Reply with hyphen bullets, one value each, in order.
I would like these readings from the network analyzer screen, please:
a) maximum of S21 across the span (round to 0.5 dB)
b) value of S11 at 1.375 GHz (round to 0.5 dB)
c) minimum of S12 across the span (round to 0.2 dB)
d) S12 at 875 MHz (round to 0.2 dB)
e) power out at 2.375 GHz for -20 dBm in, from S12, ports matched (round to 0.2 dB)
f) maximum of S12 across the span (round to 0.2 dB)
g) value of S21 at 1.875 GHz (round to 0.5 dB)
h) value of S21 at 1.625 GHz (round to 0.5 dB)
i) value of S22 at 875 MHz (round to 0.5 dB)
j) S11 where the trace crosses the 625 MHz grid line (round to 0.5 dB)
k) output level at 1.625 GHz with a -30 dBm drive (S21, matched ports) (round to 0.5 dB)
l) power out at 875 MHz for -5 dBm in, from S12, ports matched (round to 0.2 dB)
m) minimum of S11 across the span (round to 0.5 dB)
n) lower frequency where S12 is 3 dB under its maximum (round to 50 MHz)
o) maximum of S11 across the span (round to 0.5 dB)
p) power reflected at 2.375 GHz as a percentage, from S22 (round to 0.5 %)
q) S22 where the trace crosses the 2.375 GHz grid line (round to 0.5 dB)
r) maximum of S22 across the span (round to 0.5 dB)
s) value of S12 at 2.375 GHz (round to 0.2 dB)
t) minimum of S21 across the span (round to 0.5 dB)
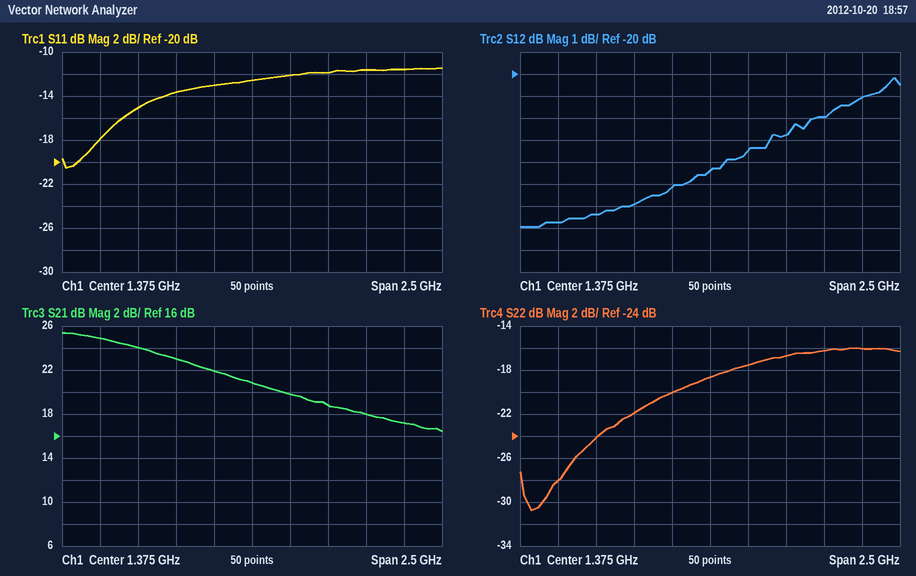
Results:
- 25.5 dB
- -12.5 dB
- -27.0 dB
- -26.0 dB
- -41.0 dBm
- -20.2 dB
- 19.0 dB
- 20.0 dB
- -22.0 dB
- -15.0 dB
- -10.0 dBm
- -31.0 dBm
- -20.5 dB
- 1.75 GHz
- -11.5 dB
- 2.5 %
- -16.0 dB
- -16.0 dB
- -21.0 dB
- 16.5 dB
